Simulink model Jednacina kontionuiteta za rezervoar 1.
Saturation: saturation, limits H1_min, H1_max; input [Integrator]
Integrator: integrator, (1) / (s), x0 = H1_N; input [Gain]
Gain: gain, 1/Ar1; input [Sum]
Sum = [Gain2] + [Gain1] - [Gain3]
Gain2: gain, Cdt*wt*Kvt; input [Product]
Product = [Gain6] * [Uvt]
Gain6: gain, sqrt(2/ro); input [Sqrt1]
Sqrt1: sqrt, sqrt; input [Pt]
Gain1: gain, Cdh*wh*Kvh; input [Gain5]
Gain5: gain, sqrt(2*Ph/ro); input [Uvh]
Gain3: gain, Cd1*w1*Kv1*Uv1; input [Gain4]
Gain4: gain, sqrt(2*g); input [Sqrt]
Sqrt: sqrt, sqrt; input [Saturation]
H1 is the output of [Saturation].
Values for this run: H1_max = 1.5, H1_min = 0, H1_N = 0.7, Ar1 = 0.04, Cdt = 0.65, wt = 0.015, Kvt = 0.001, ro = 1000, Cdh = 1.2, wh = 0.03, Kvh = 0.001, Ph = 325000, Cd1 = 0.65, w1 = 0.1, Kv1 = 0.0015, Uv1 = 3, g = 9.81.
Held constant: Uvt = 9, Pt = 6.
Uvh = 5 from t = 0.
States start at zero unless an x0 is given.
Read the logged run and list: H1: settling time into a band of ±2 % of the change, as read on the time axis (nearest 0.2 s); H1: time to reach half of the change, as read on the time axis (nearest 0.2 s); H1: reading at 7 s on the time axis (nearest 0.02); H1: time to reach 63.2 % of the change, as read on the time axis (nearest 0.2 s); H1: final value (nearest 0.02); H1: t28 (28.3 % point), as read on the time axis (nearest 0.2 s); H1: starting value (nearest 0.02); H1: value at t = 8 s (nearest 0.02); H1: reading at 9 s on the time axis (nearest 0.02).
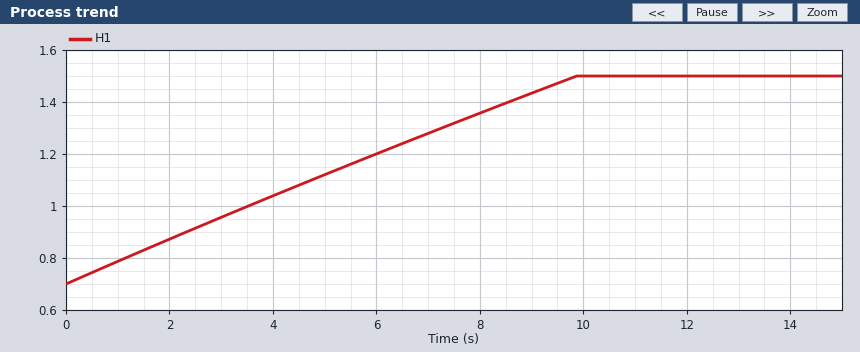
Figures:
9.6 s
4.8 s
1.28
6.0 s
1.50
2.6 s
0.70
1.36
1.44
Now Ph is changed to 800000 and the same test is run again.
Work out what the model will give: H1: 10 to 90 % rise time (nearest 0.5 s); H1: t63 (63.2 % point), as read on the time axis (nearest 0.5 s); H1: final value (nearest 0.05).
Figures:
4.5 s
3.5 s
1.50
